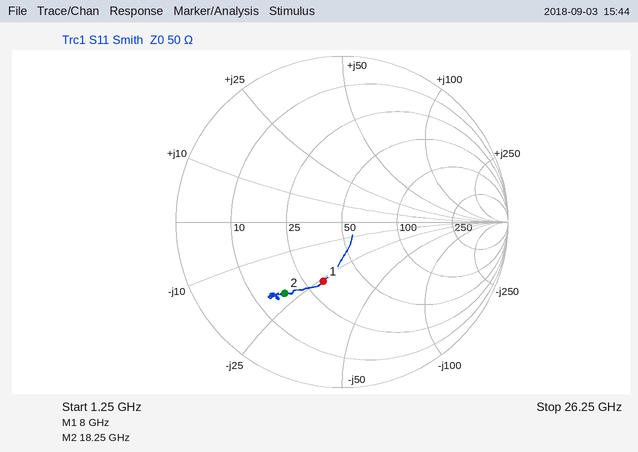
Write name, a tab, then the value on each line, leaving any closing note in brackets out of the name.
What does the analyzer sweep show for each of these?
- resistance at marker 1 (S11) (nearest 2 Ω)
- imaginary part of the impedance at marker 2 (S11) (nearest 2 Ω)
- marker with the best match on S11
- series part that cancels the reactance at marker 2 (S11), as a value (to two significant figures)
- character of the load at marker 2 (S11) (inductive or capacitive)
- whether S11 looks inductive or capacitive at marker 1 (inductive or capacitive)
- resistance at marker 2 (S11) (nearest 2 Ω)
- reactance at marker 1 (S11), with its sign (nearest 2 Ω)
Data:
resistance at marker 1 (S11)	32 Ω
imaginary part of the impedance at marker 2 (S11)	-22 Ω
marker with the best match on S11	marker 1
series part that cancels the reactance at marker 2 (S11), as a value	190 pH
character of the load at marker 2 (S11)	capacitive
whether S11 looks inductive or capacitive at marker 1	capacitive
resistance at marker 2 (S11)	18 Ω
reactance at marker 1 (S11), with its sign	-26 Ω
